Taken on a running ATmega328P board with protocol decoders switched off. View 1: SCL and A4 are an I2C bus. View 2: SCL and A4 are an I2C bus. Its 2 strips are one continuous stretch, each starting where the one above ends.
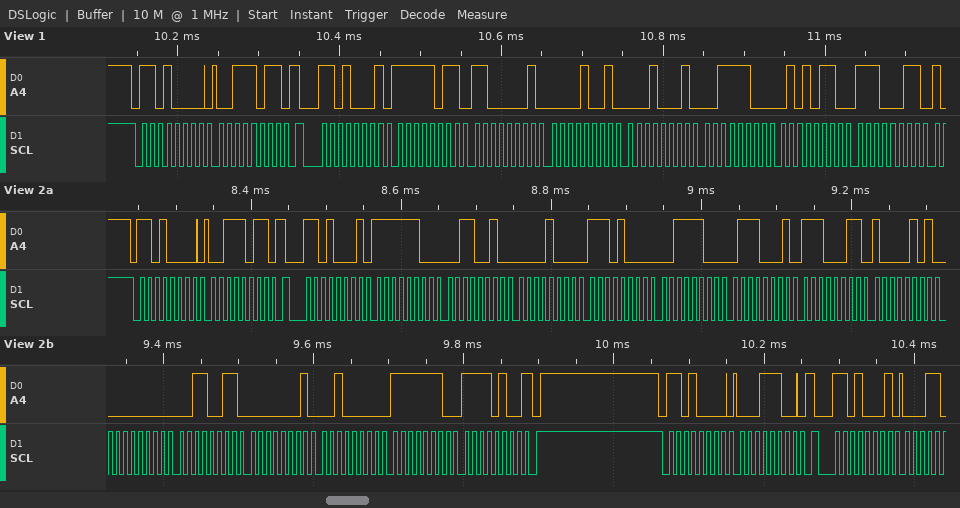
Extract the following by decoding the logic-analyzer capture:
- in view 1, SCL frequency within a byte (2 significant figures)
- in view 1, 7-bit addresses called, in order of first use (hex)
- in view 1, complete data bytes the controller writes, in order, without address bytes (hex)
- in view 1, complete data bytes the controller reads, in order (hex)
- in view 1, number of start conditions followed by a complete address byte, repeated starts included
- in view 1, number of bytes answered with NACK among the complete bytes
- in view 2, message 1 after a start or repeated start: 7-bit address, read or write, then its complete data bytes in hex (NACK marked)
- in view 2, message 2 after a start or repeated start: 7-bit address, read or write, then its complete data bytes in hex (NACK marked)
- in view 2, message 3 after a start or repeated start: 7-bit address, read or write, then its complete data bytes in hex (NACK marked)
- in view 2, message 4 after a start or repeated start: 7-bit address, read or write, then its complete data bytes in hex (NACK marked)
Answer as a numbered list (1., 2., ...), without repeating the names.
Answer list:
1. 100 kHz
2. 0x68
3. 3B
4. FB C1 09 11 3C 56 E3
5. 2
6. 0
7. 0x68 write: 3B
8. 0x68 read: FC 32 08 E8 3C 71 E3 85 00 33 01 20 FE F4 NACK
9. 0x68 write: 1C
10. 0x68 read
